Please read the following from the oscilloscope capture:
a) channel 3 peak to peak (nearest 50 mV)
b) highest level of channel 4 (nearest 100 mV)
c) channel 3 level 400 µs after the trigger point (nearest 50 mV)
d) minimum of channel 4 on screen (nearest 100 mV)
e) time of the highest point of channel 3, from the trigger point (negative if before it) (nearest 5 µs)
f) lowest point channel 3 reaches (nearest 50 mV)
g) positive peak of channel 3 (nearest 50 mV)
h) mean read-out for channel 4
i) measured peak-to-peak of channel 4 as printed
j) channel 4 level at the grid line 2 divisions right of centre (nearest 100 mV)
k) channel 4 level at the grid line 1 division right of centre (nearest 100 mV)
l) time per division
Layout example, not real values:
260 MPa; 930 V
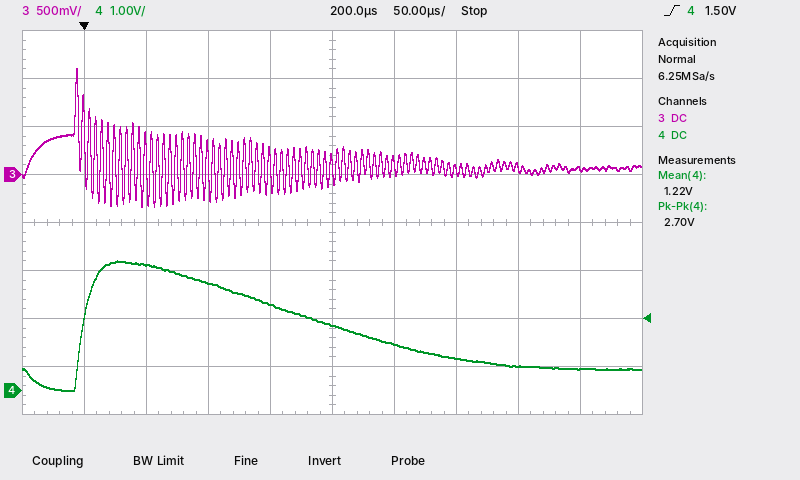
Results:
1.45 V; 2.7 V; 50 mV; 0.0 V; -5 µs; -350 mV; 1.10 V; 1.22 V; 2.70 V; 700 mV; 1.0 V; 50 µs
